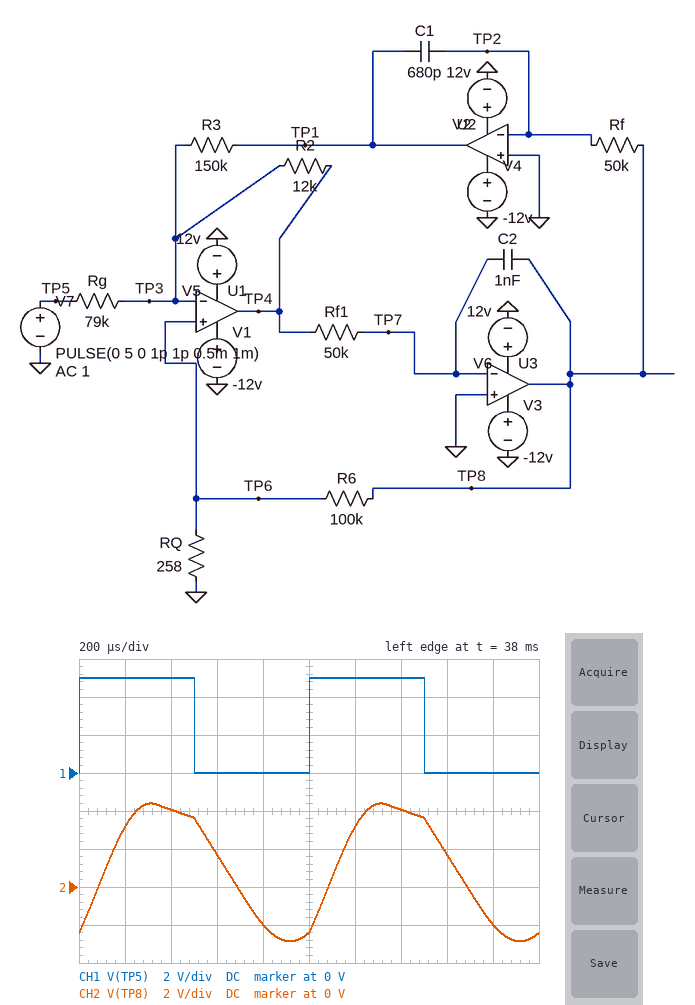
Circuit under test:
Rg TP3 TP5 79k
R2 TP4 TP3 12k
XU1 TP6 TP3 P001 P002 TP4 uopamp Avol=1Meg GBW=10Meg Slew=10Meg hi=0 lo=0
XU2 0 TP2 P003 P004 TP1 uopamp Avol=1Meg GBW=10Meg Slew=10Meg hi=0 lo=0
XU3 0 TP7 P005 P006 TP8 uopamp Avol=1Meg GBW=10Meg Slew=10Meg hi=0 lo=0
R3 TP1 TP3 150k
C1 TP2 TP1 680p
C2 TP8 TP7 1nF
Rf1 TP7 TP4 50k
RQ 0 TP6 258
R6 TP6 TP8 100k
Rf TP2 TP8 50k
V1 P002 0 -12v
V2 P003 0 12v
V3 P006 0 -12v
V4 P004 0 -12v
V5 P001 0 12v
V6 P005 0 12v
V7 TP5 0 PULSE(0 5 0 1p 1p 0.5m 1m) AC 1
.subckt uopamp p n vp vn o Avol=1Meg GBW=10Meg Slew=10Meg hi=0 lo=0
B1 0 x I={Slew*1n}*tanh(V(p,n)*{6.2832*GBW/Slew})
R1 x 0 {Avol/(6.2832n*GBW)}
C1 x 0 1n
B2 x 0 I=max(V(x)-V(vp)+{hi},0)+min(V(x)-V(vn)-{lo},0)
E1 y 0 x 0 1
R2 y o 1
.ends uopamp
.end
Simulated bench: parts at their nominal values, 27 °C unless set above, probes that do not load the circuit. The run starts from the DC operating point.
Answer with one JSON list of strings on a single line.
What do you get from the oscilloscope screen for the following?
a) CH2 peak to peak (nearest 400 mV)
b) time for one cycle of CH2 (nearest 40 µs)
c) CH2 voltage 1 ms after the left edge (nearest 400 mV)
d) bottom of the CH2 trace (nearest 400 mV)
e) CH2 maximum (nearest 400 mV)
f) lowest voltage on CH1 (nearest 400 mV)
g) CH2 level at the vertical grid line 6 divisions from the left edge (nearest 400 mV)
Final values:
["7.2 V", "1.00 ms", "-2.4 V", "-2.8 V", "4.4 V", "0 V", "3.2 V"]
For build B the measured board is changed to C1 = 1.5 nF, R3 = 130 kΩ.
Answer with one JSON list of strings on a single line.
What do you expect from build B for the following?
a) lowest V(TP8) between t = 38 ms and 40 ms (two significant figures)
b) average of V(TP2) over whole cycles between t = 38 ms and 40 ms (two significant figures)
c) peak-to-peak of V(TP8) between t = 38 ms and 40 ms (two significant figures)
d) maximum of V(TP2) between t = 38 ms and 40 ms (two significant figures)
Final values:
["-4.3 V", "36 mV", "8.8 V", "470 mV"]
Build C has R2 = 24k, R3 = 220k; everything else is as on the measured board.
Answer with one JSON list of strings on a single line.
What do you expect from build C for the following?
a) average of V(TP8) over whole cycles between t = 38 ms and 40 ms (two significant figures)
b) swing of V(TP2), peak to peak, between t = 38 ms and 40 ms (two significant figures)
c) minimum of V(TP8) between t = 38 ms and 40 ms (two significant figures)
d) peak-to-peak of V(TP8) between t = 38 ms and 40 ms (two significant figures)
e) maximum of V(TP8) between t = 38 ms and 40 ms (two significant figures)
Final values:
["2.4 V", "6.6 V", "-3.4 V", "10 V", "6.8 V"]
